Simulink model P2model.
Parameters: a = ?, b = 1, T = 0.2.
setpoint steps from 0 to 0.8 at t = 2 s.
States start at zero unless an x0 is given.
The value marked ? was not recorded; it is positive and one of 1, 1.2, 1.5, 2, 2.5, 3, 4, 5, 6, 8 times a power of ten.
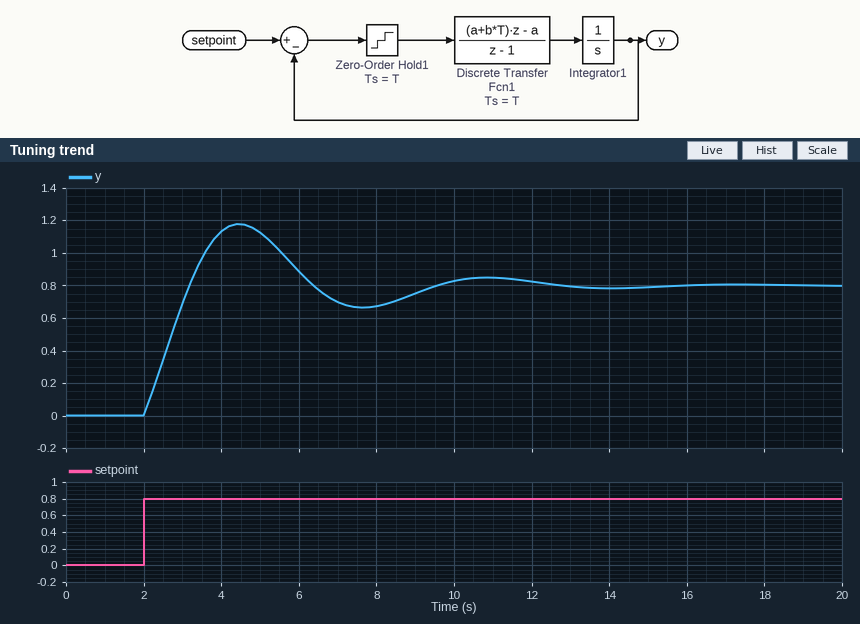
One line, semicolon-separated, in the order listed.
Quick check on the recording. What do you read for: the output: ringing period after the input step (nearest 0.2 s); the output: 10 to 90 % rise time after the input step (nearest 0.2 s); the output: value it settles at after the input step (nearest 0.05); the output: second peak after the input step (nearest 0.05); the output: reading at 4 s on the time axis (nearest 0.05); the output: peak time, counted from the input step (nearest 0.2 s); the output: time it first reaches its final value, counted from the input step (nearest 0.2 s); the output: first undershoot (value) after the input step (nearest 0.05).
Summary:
6.4 s; 1.0 s; 0.80; 0.85; 1.15; 2.4 s; 1.2 s; 0.65
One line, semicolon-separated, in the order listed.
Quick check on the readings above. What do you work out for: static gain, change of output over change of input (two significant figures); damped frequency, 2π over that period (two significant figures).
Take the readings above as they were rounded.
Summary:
1.0; 0.98 rad/s
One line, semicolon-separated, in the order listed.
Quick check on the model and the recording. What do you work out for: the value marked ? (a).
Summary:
0.6
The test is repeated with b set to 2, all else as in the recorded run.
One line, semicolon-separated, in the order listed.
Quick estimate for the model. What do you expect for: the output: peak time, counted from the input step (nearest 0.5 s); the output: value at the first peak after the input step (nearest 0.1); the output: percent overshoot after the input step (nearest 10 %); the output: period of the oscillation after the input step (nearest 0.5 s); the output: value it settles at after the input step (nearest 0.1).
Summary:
2.0 s; 1.3; 60 %; 4.5 s; 0.8
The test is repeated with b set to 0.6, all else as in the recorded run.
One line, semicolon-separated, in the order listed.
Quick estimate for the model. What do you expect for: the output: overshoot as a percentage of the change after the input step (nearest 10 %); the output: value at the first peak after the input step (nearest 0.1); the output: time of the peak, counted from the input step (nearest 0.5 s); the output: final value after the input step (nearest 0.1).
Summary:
40 %; 1.1; 3.0 s; 0.8
